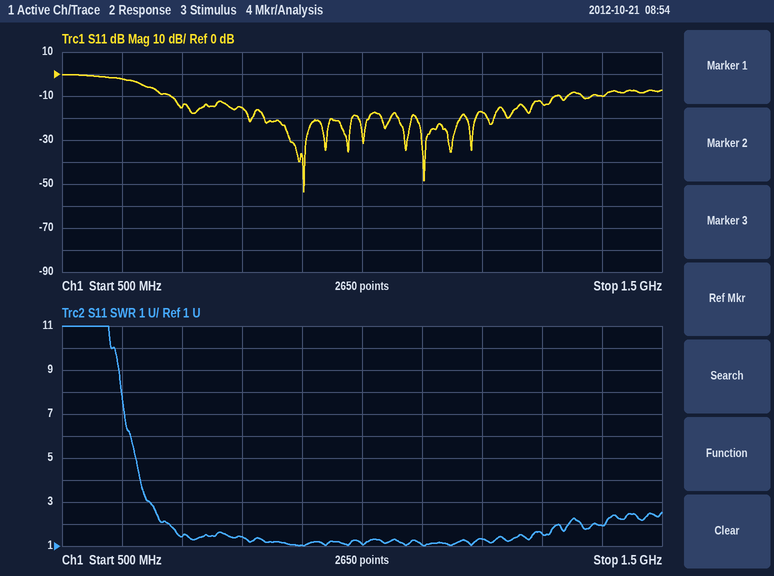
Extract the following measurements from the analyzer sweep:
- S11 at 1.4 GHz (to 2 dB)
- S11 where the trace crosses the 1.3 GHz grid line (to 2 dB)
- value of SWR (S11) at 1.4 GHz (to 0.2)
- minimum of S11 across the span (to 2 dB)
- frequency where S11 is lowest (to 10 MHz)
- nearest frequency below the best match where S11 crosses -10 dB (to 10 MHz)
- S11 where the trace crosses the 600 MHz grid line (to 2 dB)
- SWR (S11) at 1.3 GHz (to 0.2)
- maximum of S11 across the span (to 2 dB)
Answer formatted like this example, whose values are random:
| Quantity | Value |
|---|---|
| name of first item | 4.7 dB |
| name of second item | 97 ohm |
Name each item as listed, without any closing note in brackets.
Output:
| Quantity | Value |
|---|---|
| S11 at 1.4 GHz | -10 dB |
| S11 where the trace crosses the 1.3 GHz grid line | -14 dB |
| value of SWR (S11) at 1.4 GHz | 2.0 |
| minimum of S11 across the span | -54 dB |
| frequency where S11 is lowest | 900 MHz |
| nearest frequency below the best match where S11 crosses -10 dB | 680 MHz |
| S11 where the trace crosses the 600 MHz grid line | -2 dB |
| SWR (S11) at 1.3 GHz | 1.6 |
| maximum of S11 across the span | 0 dB |
